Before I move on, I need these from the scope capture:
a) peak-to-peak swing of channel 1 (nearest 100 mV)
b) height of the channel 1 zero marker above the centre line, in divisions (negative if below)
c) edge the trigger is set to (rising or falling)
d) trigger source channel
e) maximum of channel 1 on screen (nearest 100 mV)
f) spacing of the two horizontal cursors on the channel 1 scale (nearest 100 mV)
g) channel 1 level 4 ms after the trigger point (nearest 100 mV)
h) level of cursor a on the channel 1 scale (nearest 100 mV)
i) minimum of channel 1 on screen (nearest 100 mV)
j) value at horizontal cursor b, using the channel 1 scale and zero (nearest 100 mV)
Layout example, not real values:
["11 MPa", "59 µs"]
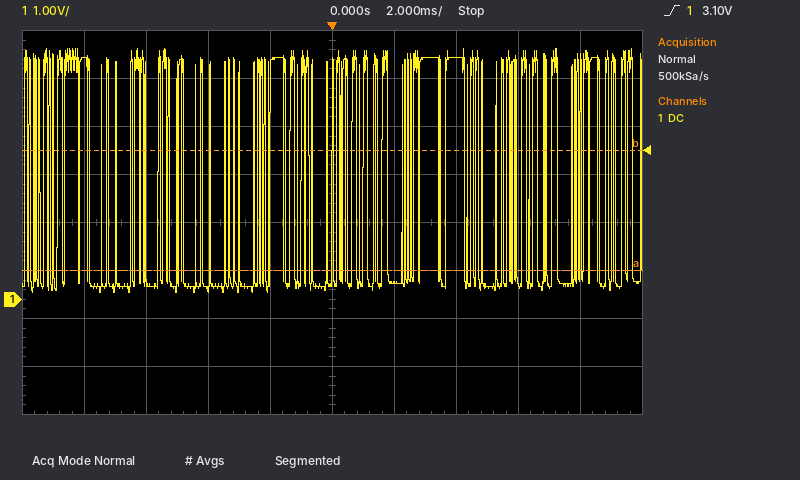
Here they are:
["5.1 V", "-1.6 div", "rising", "channel 1", "5.2 V", "2.5 V", "5.0 V", "600 mV", "100 mV", "3.1 V"]
